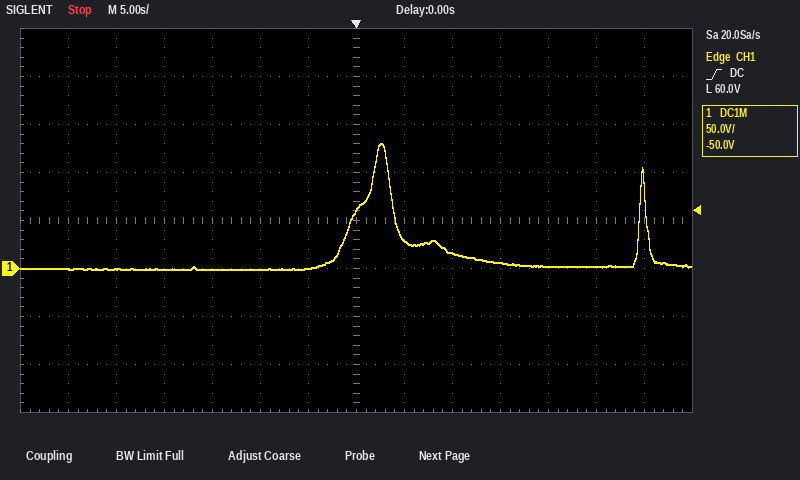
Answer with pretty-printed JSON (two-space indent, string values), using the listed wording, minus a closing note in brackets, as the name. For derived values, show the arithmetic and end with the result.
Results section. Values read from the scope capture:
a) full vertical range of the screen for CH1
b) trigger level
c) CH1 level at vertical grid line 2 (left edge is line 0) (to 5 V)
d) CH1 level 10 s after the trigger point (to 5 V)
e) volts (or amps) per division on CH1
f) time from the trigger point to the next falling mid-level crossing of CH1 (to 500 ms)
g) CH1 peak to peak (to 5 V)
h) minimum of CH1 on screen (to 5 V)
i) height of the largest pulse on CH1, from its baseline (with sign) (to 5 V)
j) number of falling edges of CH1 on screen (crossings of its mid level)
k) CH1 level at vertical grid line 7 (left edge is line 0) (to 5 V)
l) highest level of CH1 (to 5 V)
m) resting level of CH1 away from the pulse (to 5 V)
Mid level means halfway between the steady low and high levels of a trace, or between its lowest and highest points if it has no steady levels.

{
  "full vertical range of the screen for CH1": "400 V",
  "trigger level": "60.0 V",
  "CH1 level at vertical grid line 2 (left edge is line 0)": "0 V",
  "CH1 level 10 s after the trigger point": "15 V",
  "volts (or amps) per division on CH1": "50 V",
  "time from the trigger point to the next falling mid-level crossing of CH1": "4.0 s",
  "CH1 peak to peak": "130 V − (0 V) = 130 V",
  "minimum of CH1 on screen": "0 V",
  "height of the largest pulse on CH1, from its baseline (with sign)": "130 V − (0 V) = +130 V",
  "number of falling edges of CH1 on screen": "2",
  "CH1 level at vertical grid line 7 (left edge is line 0)": "60 V",
  "highest level of CH1": "130 V",
  "resting level of CH1 away from the pulse": "0 V"
}
